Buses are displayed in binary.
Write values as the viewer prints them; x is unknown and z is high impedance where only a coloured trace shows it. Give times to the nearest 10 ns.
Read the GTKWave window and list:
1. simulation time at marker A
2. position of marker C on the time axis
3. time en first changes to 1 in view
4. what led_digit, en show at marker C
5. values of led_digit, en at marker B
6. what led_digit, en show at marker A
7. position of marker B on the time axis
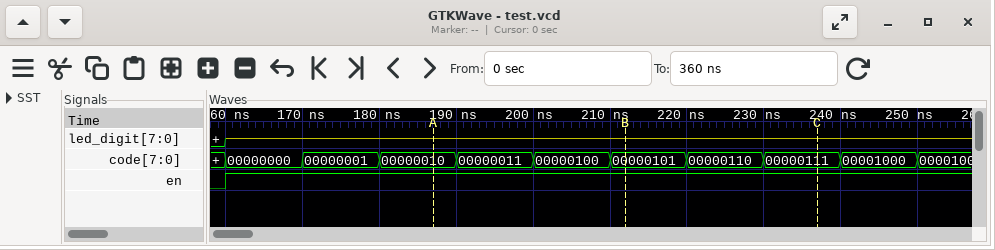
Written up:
190 ns
240 ns
160 ns
led_digit=z, en=1
led_digit=z, en=1
led_digit=z, en=1
210 ns
